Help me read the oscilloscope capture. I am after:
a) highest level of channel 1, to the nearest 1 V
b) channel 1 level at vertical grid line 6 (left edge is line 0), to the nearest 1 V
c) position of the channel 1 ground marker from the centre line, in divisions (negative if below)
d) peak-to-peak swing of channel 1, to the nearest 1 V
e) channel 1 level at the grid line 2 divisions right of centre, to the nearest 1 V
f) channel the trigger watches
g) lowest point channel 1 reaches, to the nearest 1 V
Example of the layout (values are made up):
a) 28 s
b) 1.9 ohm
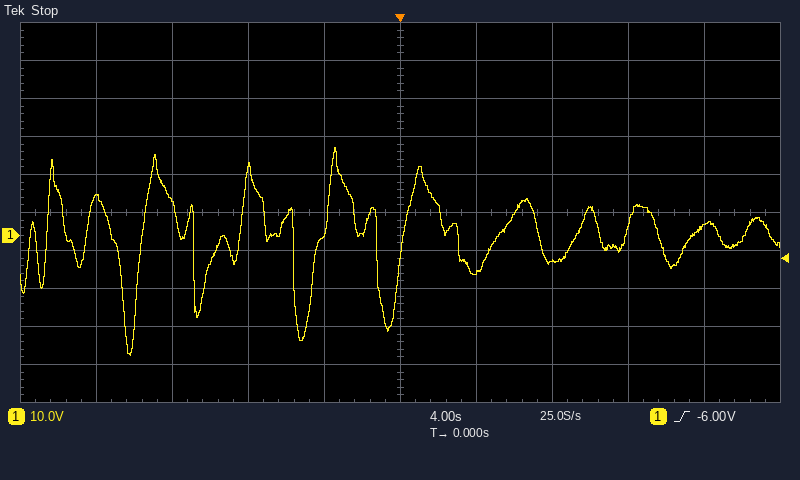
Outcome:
a) 23 V
b) -10 V
c) -0.6 div
d) 55 V
e) -7 V
f) channel 1
g) -32 V
